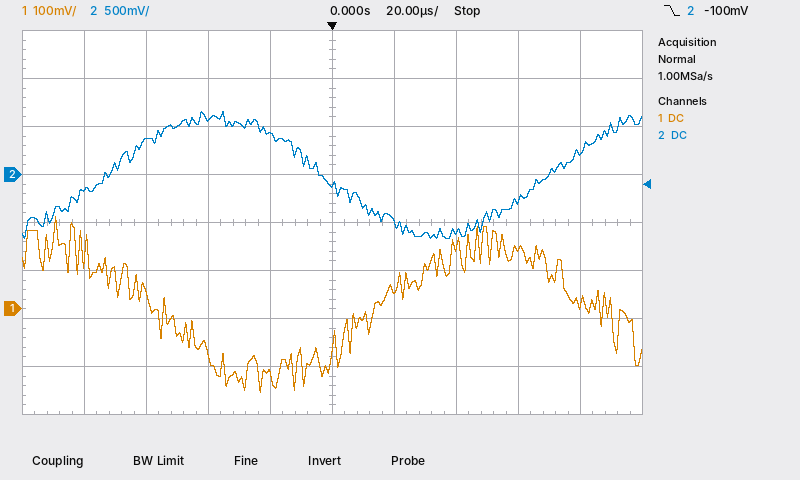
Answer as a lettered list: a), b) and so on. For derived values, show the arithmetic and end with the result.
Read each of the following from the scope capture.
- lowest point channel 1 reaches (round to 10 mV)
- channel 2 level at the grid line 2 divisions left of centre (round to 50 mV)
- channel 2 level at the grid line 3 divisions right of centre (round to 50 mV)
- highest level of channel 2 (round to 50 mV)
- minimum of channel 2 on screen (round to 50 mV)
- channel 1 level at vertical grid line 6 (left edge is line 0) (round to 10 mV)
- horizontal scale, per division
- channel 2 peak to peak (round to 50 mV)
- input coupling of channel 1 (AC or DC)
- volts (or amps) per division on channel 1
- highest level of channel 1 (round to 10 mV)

a) -170 mV
b) 600 mV
c) -250 mV
d) 650 mV
e) -650 mV
f) 40 mV
g) 20 µs
h) 650 mV − (-650 mV) = 1.30 V
i) DC
j) 100 mV
k) 190 mV
